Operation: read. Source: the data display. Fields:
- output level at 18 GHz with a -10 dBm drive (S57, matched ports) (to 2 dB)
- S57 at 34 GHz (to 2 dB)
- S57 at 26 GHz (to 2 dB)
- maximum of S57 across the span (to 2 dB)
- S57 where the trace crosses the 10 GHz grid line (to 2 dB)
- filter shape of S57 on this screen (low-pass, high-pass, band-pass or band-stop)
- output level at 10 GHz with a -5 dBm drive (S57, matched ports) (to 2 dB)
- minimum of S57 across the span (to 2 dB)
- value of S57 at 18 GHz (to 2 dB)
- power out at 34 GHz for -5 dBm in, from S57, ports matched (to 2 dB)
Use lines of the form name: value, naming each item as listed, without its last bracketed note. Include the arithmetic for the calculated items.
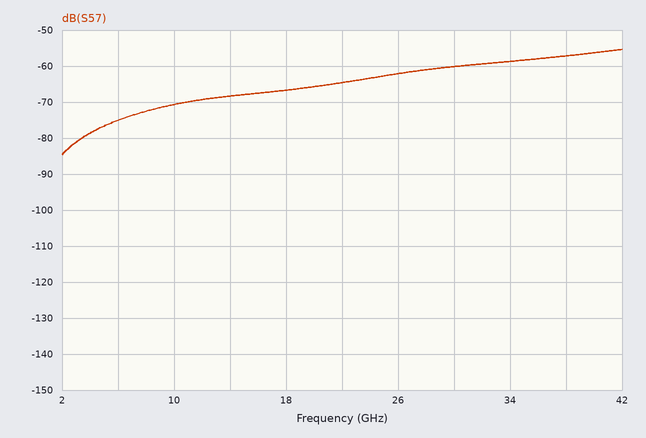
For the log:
output level at 18 GHz with a -10 dBm drive (S57, matched ports): -10 dBm + (-66 dB) = -76 dBm
S57 at 34 GHz: -58 dB
S57 at 26 GHz: -62 dB
maximum of S57 across the span: -56 dB
S57 where the trace crosses the 10 GHz grid line: -70 dB
filter shape of S57 on this screen: high-pass
output level at 10 GHz with a -5 dBm drive (S57, matched ports): -5 dBm + (-70 dB) = -76 dBm
minimum of S57 across the span: -84 dB
value of S57 at 18 GHz: -66 dB
power out at 34 GHz for -5 dBm in, from S57, ports matched: -5 dBm + (-58 dB) = -64 dBm
